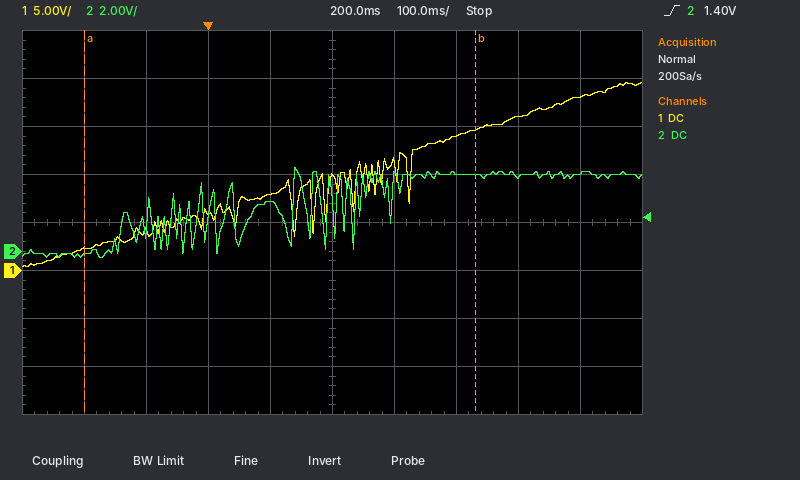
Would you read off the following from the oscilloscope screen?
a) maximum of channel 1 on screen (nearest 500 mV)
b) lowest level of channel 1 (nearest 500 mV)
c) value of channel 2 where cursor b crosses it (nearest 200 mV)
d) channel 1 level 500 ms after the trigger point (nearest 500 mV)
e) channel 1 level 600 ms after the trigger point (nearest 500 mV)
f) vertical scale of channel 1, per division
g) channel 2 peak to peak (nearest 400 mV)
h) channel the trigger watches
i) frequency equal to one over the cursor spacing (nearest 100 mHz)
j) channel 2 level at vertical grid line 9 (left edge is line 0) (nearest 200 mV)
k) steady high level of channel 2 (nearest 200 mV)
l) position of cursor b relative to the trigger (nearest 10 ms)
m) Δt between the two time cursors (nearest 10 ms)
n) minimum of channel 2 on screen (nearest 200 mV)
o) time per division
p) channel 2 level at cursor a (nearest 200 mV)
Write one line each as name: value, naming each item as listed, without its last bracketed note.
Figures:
maximum of channel 1 on screen: 19.5 V
lowest level of channel 1: 500 mV
value of channel 2 where cursor b crosses it: 3.2 V
channel 1 level 500 ms after the trigger point: 16.0 V
channel 1 level 600 ms after the trigger point: 18.0 V
vertical scale of channel 1, per division: 5 V
channel 2 peak to peak: 3.6 V
channel the trigger watches: channel 2
frequency equal to one over the cursor spacing: 1.6 Hz
channel 2 level at vertical grid line 9 (left edge is line 0): 3.2 V
steady high level of channel 2: 3.2 V
position of cursor b relative to the trigger: +430 ms
Δt between the two time cursors: 630 ms
minimum of channel 2 on screen: -200 mV
time per division: 100 ms
channel 2 level at cursor a: -200 mV
